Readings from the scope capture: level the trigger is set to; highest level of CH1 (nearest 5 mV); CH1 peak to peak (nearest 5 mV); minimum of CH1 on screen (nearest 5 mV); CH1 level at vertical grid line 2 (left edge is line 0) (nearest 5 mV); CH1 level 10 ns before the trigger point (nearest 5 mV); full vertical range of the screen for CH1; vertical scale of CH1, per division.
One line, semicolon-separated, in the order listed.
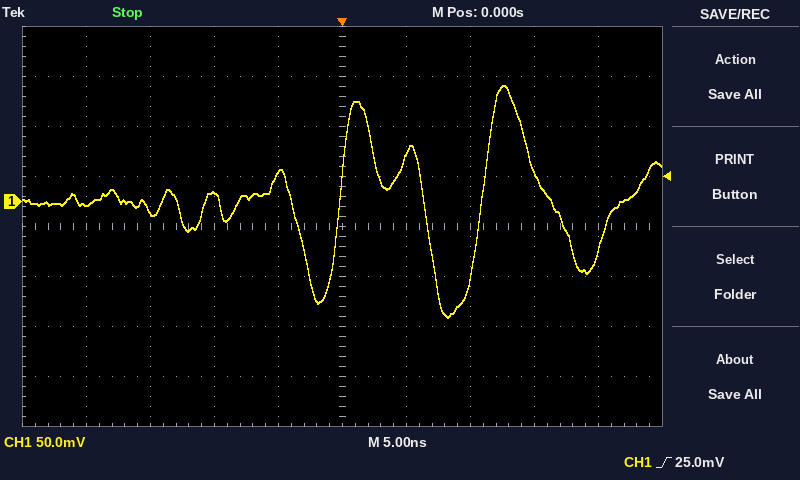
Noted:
25.0 mV; 115 mV; 230 mV; -115 mV; -10 mV; 10 mV; 400 mV; 50 mV
